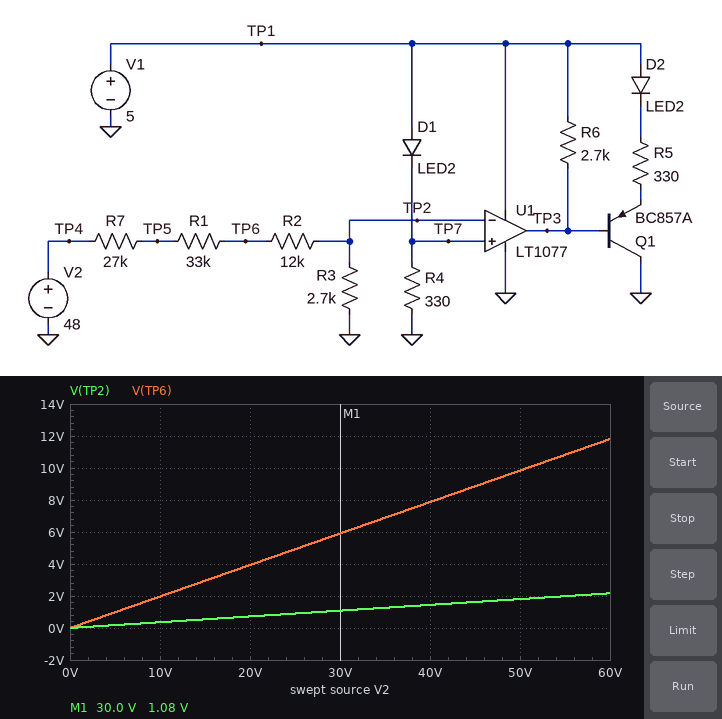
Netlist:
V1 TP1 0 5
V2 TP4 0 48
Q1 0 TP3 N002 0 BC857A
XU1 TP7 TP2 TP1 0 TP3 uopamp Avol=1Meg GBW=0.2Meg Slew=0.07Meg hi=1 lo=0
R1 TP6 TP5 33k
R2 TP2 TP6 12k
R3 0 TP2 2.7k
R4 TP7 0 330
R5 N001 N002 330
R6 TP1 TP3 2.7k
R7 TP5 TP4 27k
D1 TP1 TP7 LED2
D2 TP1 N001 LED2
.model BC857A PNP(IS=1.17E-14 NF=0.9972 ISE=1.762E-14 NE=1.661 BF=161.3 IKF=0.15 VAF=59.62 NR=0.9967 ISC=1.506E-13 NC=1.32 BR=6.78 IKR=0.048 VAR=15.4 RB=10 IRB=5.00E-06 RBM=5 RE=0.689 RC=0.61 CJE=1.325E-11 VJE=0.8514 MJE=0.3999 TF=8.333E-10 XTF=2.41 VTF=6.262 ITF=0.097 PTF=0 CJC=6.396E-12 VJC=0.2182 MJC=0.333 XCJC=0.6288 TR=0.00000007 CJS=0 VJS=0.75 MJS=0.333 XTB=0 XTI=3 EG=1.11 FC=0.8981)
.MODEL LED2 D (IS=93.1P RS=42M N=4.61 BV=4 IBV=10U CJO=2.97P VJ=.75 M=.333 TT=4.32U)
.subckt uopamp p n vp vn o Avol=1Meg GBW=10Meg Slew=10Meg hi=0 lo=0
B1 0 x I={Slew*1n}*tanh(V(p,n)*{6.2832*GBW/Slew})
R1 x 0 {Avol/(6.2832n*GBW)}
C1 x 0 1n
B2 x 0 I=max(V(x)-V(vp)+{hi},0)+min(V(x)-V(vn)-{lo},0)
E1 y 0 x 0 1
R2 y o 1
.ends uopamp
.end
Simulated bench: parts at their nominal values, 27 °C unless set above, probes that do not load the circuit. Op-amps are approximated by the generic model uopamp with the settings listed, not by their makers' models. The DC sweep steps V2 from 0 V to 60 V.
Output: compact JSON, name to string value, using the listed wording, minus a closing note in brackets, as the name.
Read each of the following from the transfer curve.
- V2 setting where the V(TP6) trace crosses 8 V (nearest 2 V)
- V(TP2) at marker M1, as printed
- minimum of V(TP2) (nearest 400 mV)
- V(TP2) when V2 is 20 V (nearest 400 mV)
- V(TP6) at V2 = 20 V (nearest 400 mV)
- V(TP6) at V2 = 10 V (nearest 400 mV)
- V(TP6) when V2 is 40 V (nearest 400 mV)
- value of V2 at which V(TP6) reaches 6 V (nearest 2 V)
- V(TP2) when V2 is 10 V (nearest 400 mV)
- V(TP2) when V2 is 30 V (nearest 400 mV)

{"V2 setting where the V(TP6) trace crosses 8 V": "40 V", "V(TP2) at marker M1, as printed": "1.08 V", "minimum of V(TP2)": "0 V", "V(TP2) when V2 is 20 V": "800 mV", "V(TP6) at V2 = 20 V": "4.0 V", "V(TP6) at V2 = 10 V": "2.0 V", "V(TP6) when V2 is 40 V": "8.0 V", "value of V2 at which V(TP6) reaches 6 V": "30 V", "V(TP2) when V2 is 10 V": "400 mV", "V(TP2) when V2 is 30 V": "1.2 V"}
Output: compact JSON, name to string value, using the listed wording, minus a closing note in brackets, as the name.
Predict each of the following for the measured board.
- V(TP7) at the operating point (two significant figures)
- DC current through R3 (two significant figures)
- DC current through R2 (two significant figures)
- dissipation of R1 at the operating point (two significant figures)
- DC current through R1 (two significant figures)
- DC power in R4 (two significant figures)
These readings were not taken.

{"V(TP7) at the operating point": "2.8 V", "DC current through R3": "640 µA", "DC current through R2": "640 µA", "dissipation of R1 at the operating point": "14 mW", "DC current through R1": "640 µA", "DC power in R4": "24 mW"}
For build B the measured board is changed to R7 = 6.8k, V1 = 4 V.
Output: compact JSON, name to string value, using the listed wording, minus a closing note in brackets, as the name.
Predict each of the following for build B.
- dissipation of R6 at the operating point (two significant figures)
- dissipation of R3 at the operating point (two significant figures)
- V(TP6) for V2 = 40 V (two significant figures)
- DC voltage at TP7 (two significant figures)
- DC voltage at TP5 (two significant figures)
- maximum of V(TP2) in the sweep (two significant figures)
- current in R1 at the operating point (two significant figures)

{"dissipation of R6 at the operating point": "5.9 mW", "dissipation of R3 at the operating point": "2.1 mW", "V(TP6) for V2 = 40 V": "11 V", "DC voltage at TP7": "1.9 V", "DC voltage at TP5": "42 V", "maximum of V(TP2) in the sweep": "3.0 V", "current in R1 at the operating point": "880 µA"}
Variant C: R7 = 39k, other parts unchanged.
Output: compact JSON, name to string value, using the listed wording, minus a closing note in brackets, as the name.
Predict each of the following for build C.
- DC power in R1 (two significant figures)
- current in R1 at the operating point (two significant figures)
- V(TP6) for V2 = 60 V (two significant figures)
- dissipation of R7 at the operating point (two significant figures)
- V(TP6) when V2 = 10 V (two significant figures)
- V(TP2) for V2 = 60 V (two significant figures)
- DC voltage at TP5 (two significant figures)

{"DC power in R1": "10 mW", "current in R1 at the operating point": "550 µA", "V(TP6) for V2 = 60 V": "10 V", "dissipation of R7 at the operating point": "12 mW", "V(TP6) when V2 = 10 V": "1.7 V", "V(TP2) for V2 = 60 V": "1.9 V", "DC voltage at TP5": "26 V"}
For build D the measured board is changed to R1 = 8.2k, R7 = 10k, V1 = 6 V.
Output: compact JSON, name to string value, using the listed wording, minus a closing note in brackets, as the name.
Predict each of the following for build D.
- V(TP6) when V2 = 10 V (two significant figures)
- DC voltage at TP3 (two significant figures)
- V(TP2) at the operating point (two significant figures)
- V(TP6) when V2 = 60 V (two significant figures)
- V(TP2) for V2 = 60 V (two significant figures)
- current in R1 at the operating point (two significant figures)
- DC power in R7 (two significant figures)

{"V(TP6) when V2 = 10 V": "4.5 V", "DC voltage at TP3": "2.2 mV", "V(TP2) at the operating point": "3.9 V", "V(TP6) when V2 = 60 V": "27 V", "V(TP2) for V2 = 60 V": "4.9 V", "current in R1 at the operating point": "1.5 mA", "DC power in R7": "21 mW"}
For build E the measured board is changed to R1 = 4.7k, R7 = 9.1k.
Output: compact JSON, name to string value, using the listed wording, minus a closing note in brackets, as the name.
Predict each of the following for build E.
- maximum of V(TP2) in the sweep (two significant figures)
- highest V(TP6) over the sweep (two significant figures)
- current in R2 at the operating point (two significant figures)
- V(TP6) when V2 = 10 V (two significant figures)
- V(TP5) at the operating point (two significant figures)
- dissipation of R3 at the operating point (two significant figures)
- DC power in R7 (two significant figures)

{"maximum of V(TP2) in the sweep": "5.7 V", "highest V(TP6) over the sweep": "31 V", "current in R2 at the operating point": "1.7 mA", "V(TP6) when V2 = 10 V": "5.2 V", "V(TP5) at the operating point": "33 V", "dissipation of R3 at the operating point": "7.7 mW", "DC power in R7": "26 mW"}
